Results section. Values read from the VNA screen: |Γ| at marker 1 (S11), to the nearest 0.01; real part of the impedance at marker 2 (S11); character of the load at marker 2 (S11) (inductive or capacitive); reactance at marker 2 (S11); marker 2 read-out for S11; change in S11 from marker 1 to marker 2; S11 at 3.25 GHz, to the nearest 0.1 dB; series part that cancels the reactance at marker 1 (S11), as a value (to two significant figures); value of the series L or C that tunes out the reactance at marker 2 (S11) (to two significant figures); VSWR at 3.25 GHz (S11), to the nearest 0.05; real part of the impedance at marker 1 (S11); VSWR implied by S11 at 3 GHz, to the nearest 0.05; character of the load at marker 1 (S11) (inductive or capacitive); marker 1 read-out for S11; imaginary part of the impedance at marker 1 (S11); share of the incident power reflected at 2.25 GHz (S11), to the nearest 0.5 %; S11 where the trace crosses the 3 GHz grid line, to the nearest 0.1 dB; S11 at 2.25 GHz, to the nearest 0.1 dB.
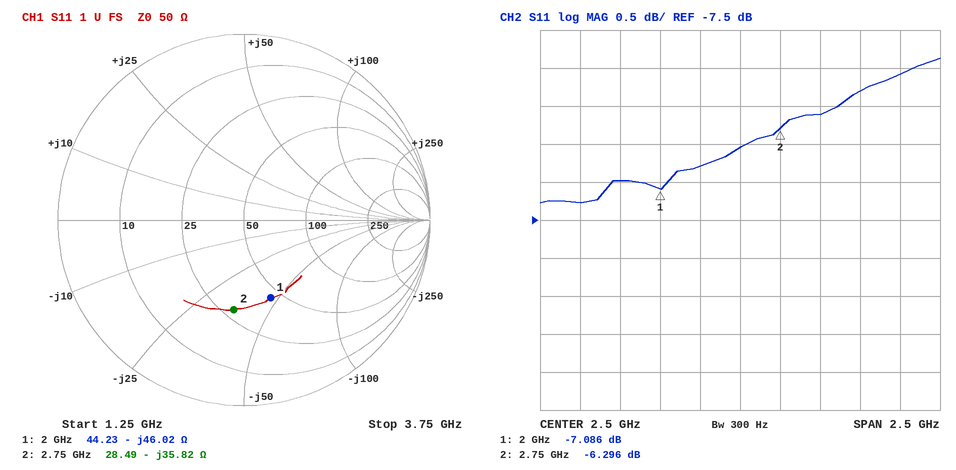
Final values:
0.44
28.49 Ω
capacitive
-35.82 Ω
-6.296 dB
0.790 dB
-5.8 dB
3.7 nH
2.1 nH
3.10
44.23 Ω
2.95
capacitive
-7.086 dB
-46.02 Ω
21.0 %
-6.1 dB
-6.8 dB
